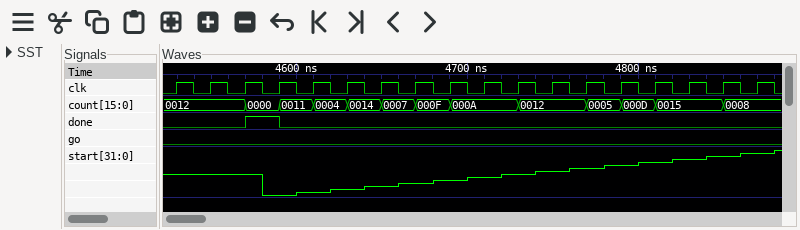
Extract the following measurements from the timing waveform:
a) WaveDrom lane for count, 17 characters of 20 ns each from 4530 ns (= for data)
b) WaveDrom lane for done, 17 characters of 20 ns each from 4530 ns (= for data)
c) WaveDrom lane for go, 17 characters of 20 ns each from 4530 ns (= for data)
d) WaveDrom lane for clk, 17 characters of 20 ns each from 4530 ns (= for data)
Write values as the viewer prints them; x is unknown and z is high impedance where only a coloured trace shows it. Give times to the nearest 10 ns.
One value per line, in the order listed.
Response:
{name: 'count', wave: '=.=======.=.===.=', data: '0012 0000 0011 0004 0014 0007 000F 000A 0012 0005 000D 0015 0008'}
{name: 'done', wave: '0.10.............'}
{name: 'go', wave: '0................'}
{name: 'clk', wave: 'p................'}
